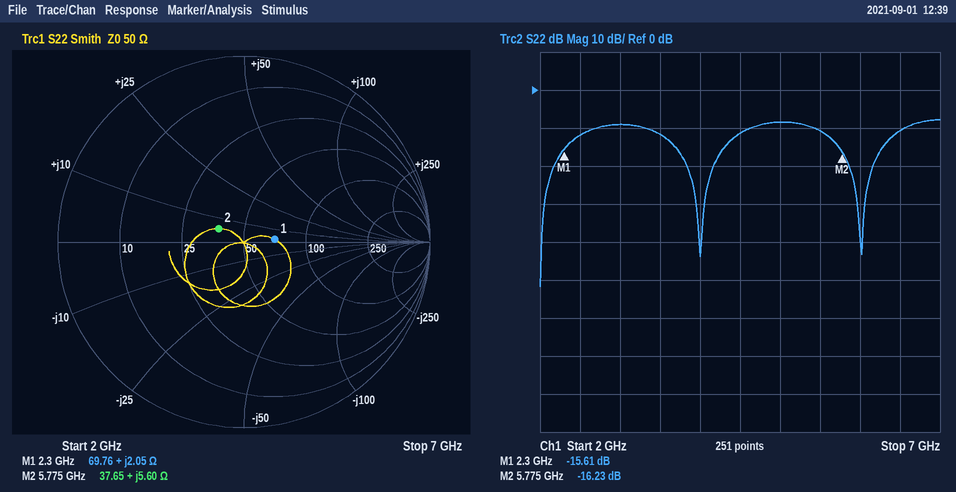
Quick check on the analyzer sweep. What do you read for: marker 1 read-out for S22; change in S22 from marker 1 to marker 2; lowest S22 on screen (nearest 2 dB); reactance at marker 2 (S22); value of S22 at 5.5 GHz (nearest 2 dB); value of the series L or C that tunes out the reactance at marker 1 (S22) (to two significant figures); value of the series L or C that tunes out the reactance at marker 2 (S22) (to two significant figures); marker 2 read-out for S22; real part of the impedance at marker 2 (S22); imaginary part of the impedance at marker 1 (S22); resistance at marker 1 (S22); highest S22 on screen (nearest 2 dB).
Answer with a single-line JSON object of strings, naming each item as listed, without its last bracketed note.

{"marker 1 read-out for S22": "-15.61 dB", "change in S22 from marker 1 to marker 2": "-0.62 dB", "lowest S22 on screen": "-52 dB", "reactance at marker 2": "+5.60 Ω", "value of S22 at 5.5 GHz": "-10 dB", "value of the series L or C that tunes out the reactance at marker 1 (S22)": "34 pF", "value of the series L or C that tunes out the reactance at marker 2 (S22)": "4.9 pF", "marker 2 read-out for S22": "-16.23 dB", "real part of the impedance at marker 2": "37.65 Ω", "imaginary part of the impedance at marker 1": "+2.05 Ω", "resistance at marker 1": "69.76 Ω", "highest S22 on screen": "-8 dB"}
